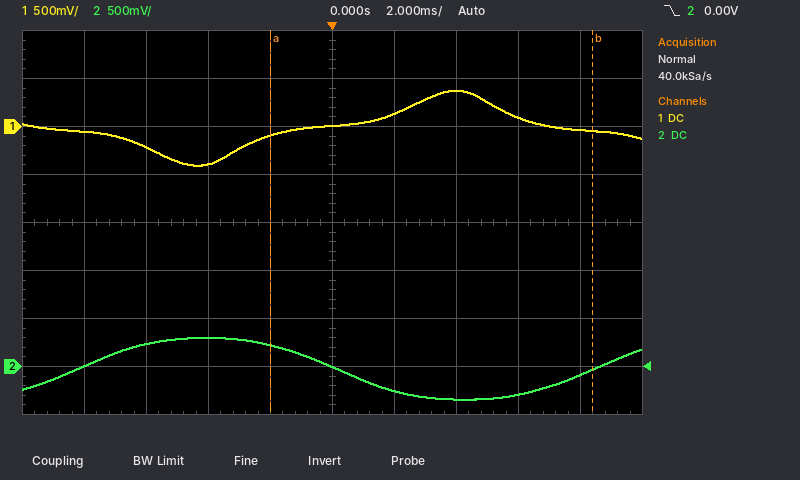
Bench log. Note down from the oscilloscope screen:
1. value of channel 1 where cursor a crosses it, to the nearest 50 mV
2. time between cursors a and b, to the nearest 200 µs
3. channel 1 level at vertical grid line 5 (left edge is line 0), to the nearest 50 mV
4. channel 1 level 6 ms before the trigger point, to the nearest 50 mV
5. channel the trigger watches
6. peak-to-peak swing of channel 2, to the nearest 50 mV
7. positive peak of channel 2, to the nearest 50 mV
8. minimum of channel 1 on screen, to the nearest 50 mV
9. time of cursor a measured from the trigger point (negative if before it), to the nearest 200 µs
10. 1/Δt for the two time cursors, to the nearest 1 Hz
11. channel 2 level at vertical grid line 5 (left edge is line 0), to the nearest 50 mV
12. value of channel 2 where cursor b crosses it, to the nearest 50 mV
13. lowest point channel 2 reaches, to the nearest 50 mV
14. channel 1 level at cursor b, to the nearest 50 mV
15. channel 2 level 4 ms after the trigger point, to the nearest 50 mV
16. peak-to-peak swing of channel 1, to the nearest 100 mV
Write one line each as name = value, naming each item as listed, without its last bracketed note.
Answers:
value of channel 1 where cursor a crosses it, to the nearest 50 mV = -100 mV
time between cursors a and b, to the nearest 200 µs = 10.4 ms
channel 1 level at vertical grid line 5 (left edge is line 0), to the nearest 50 mV = 0 mV
channel 1 level 6 ms before the trigger point, to the nearest 50 mV = -200 mV
channel the trigger watches = channel 2
peak-to-peak swing of channel 2, to the nearest 50 mV = 650 mV
positive peak of channel 2, to the nearest 50 mV = 300 mV
minimum of channel 1 on screen, to the nearest 50 mV = -400 mV
time of cursor a measured from the trigger point (negative if before it), to the nearest 200 µs = -2.0 ms
1/Δt for the two time cursors, to the nearest 1 Hz = 96 Hz
channel 2 level at vertical grid line 5 (left edge is line 0), to the nearest 50 mV = 0 mV
value of channel 2 where cursor b crosses it, to the nearest 50 mV = -50 mV
lowest point channel 2 reaches, to the nearest 50 mV = -350 mV
channel 1 level at cursor b, to the nearest 50 mV = -50 mV
channel 2 level 4 ms after the trigger point, to the nearest 50 mV = -350 mV
peak-to-peak swing of channel 1, to the nearest 100 mV = 800 mV
